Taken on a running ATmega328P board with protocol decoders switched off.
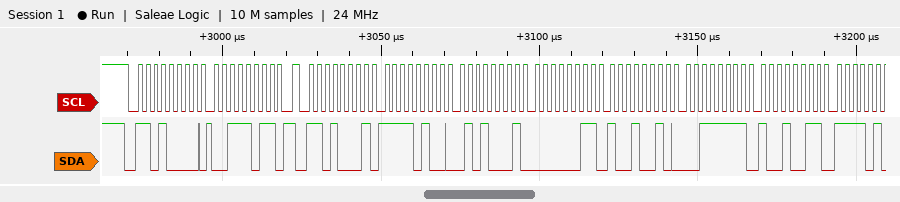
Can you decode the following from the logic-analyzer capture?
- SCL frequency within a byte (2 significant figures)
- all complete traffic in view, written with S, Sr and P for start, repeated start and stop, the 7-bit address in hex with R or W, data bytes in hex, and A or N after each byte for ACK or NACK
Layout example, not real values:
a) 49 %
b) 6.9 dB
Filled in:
a) 400 kHz
b) S 68W A 3B A Sr 68R A F4 A 51 A 03 A 92 A 3F A 93 A
